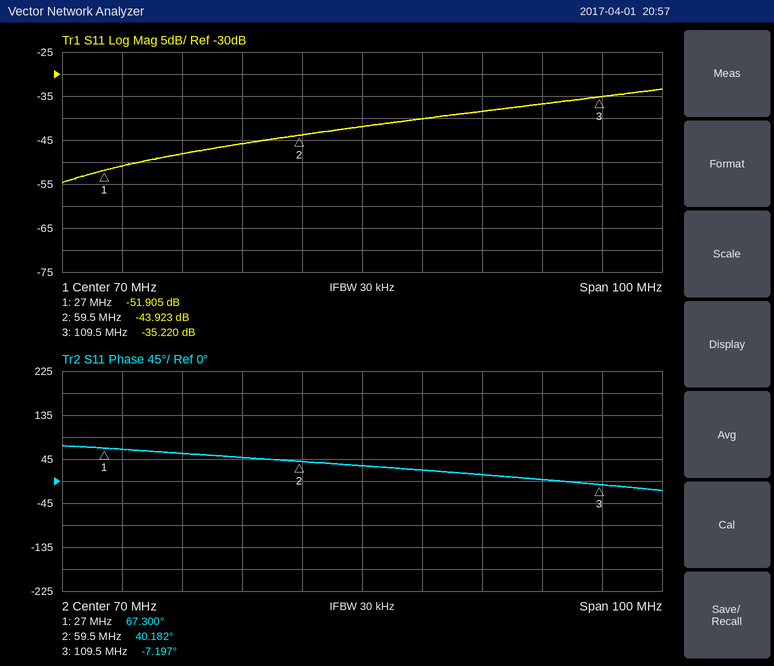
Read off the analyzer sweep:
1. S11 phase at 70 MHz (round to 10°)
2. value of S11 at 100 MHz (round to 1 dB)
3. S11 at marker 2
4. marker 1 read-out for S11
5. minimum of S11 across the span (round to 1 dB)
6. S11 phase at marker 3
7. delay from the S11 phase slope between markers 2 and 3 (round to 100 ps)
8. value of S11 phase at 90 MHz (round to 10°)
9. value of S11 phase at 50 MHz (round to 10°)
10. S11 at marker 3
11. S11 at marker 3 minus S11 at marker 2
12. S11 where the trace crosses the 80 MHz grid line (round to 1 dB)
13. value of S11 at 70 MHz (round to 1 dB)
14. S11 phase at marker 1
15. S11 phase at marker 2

30°
-37 dB
-43.923 dB
-51.905 dB
-55 dB
-7.197°
2.6 ns
10°
50°
-35.220 dB
8.703 dB
-40 dB
-42 dB
67.300°
40.182°
